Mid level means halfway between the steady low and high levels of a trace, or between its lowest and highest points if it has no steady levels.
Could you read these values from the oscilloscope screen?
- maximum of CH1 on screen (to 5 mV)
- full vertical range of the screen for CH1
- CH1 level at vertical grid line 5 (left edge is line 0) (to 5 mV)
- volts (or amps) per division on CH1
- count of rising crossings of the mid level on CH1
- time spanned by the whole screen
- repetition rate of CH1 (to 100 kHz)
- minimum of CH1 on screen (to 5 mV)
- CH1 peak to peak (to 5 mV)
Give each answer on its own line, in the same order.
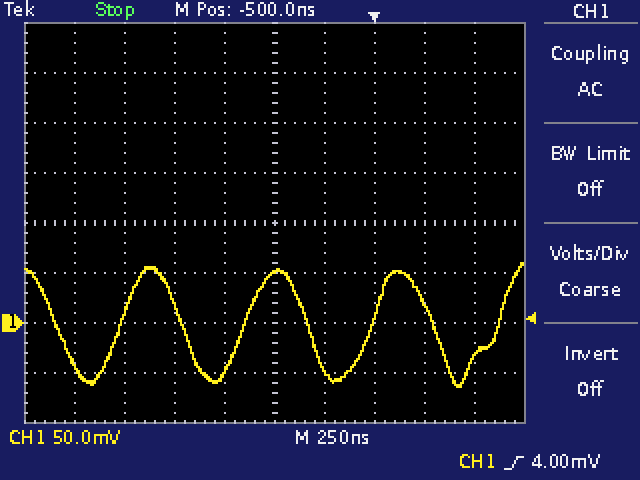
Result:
60 mV
400 mV
50 mV
50 mV
4
2.5 µs
1.6 MHz
-65 mV
125 mV
